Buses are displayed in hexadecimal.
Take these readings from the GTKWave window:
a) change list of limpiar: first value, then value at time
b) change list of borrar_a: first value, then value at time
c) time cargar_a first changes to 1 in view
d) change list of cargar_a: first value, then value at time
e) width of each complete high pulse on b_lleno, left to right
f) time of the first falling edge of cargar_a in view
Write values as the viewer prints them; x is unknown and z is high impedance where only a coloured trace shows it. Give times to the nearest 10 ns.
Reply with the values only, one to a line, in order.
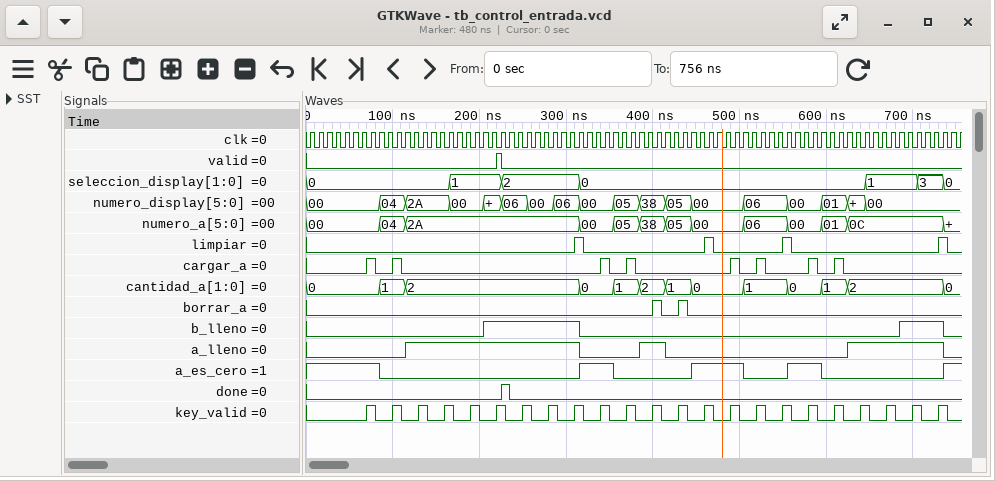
0, 1 at 310 ns, 0 at 320 ns, 1 at 460 ns, 0 at 470 ns, 1 at 550 ns, 0 at 560 ns, 1 at 730 ns, 0 at 740 ns
0, 1 at 400 ns, 0 at 410 ns, 1 at 430 ns, 0 at 440 ns
70 ns
0, 1 at 70 ns, 0 at 80 ns, 1 at 100 ns, 0 at 110 ns, 1 at 340 ns, 0 at 350 ns, 1 at 370 ns, 0 at 380 ns, 1 at 490 ns, 0 at 500 ns, 1 at 520 ns, 0 at 530 ns, 1 at 580 ns, 0 at 590 ns, 1 at 610 ns, 0 at 620 ns
110 ns, 50 ns
80 ns
